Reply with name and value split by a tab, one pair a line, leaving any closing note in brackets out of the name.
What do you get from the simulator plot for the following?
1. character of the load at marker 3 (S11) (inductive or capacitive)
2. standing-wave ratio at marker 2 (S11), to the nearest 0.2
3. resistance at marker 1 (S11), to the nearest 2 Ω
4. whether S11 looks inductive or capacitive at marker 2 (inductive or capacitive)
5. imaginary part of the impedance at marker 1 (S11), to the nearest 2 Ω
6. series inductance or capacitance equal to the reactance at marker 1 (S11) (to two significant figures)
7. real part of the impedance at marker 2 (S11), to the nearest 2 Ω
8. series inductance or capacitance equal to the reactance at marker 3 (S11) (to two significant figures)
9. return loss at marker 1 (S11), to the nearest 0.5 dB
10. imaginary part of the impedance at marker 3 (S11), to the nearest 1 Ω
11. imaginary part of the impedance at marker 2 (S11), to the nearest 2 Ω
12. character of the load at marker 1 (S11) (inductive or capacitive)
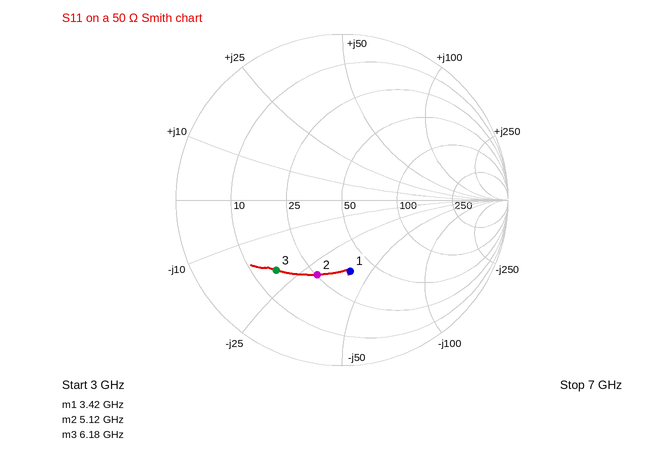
character of the load at marker 3 (S11)	capacitive
standing-wave ratio at marker 2 (S11), to the nearest 0.2	2.8
resistance at marker 1 (S11), to the nearest 2 Ω	38 Ω
whether S11 looks inductive or capacitive at marker 2	capacitive
imaginary part of the impedance at marker 1 (S11), to the nearest 2 Ω	-40 Ω
series inductance or capacitance equal to the reactance at marker 1 (S11)	1.2 pF
real part of the impedance at marker 2 (S11), to the nearest 2 Ω	26 Ω
series inductance or capacitance equal to the reactance at marker 3 (S11)	1.3 pF
return loss at marker 1 (S11), to the nearest 0.5 dB	7.5 dB
imaginary part of the impedance at marker 3 (S11), to the nearest 1 Ω	-20 Ω
imaginary part of the impedance at marker 2 (S11), to the nearest 2 Ω	-30 Ω
character of the load at marker 1 (S11)	capacitive
